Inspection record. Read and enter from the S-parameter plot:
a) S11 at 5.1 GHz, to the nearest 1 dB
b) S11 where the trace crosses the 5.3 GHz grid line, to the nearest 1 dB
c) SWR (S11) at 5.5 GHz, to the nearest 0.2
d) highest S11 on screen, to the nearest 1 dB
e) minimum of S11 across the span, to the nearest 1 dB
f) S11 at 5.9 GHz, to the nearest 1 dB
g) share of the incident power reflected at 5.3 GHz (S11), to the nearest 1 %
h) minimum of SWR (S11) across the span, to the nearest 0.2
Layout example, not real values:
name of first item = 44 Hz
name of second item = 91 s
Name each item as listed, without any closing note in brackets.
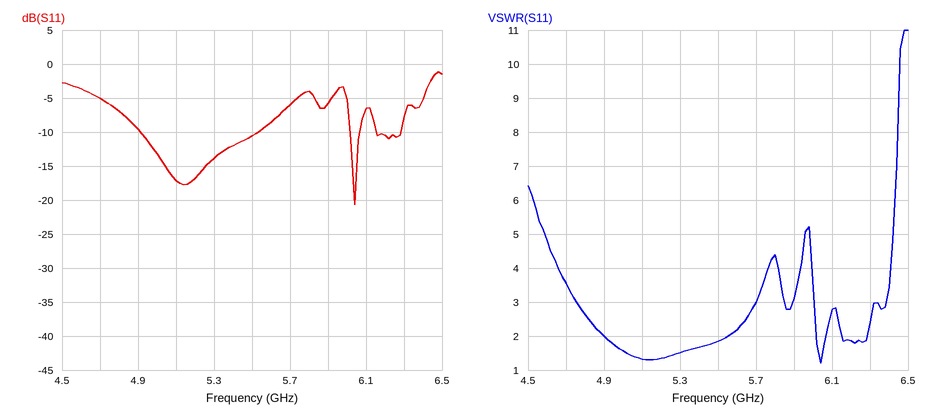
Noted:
S11 at 5.1 GHz, to the nearest 1 dB = -17 dB
S11 where the trace crosses the 5.3 GHz grid line, to the nearest 1 dB = -14 dB
SWR (S11) at 5.5 GHz, to the nearest 0.2 = 1.8
highest S11 on screen, to the nearest 1 dB = -1 dB
minimum of S11 across the span, to the nearest 1 dB = -21 dB
S11 at 5.9 GHz, to the nearest 1 dB = -6 dB
share of the incident power reflected at 5.3 GHz (S11), to the nearest 1 % = 4 %
minimum of SWR (S11) across the span, to the nearest 0.2 = 1.2
